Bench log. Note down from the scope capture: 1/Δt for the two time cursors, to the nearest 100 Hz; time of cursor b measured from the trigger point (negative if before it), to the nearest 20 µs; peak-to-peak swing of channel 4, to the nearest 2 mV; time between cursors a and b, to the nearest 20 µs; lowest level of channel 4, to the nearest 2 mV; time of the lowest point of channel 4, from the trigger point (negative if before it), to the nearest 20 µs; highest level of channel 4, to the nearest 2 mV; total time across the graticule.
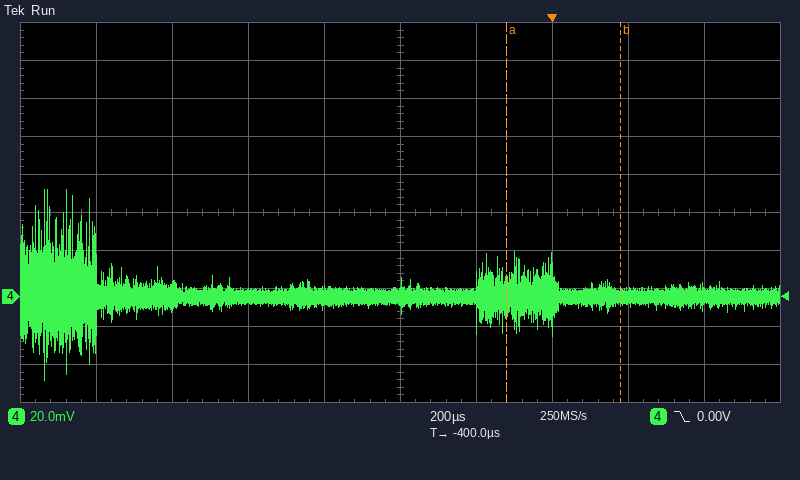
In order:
3.3 kHz
+180 µs
100 mV
300 µs
-44 mV
-1.34 ms
56 mV
2 ms
